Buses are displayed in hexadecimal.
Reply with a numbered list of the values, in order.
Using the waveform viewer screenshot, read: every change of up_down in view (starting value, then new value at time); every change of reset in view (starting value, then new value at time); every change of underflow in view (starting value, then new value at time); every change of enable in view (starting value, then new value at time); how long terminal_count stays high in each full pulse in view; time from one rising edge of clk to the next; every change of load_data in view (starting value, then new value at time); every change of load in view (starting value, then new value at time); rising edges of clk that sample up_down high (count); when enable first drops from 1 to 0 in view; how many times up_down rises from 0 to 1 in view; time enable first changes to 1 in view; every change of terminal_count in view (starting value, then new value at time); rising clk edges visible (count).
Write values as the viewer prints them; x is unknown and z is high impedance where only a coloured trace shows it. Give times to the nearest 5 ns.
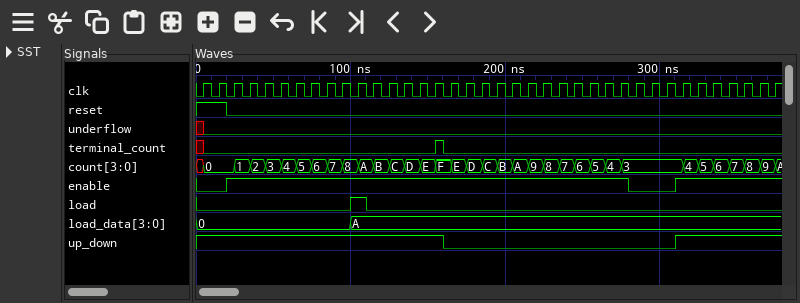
1. 1, 0 at 160 ns, 1 at 310 ns
2. 1, 0 at 20 ns
3. x, 0 at 5 ns
4. 0, 1 at 20 ns, 0 at 280 ns, 1 at 310 ns
5. 5 ns
6. 10 ns
7. 0, A at 100 ns
8. 0, 1 at 100 ns, 0 at 110 ns
9. 23
10. 280 ns
11. 1
12. 20 ns
13. x, 0 at 5 ns, 1 at 155 ns, 0 at 160 ns
14. 38
